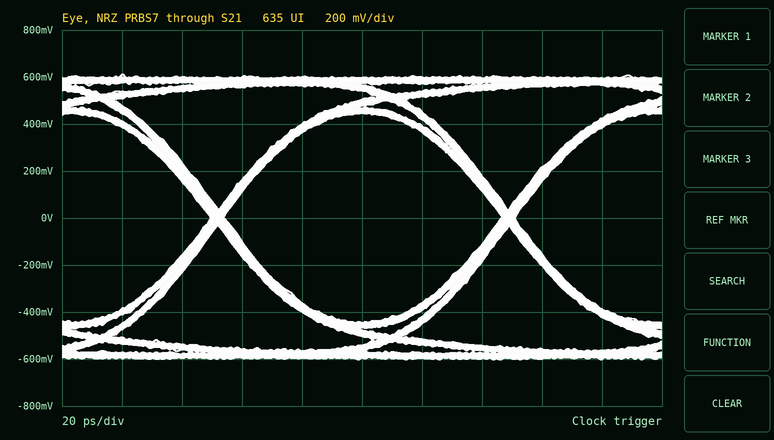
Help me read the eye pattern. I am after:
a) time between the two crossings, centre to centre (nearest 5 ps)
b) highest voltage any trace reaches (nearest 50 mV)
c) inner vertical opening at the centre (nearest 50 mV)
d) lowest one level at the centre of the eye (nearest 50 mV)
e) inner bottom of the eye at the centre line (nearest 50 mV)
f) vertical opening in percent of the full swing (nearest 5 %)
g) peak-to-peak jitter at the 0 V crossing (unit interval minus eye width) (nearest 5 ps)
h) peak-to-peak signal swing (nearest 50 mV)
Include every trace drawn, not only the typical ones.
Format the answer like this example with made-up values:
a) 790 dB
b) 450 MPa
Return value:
a) 95 ps
b) 600 mV
c) 900 mV
d) 450 mV
e) -450 mV
f) 75 %
g) 5 ps
h) 1.20 V
